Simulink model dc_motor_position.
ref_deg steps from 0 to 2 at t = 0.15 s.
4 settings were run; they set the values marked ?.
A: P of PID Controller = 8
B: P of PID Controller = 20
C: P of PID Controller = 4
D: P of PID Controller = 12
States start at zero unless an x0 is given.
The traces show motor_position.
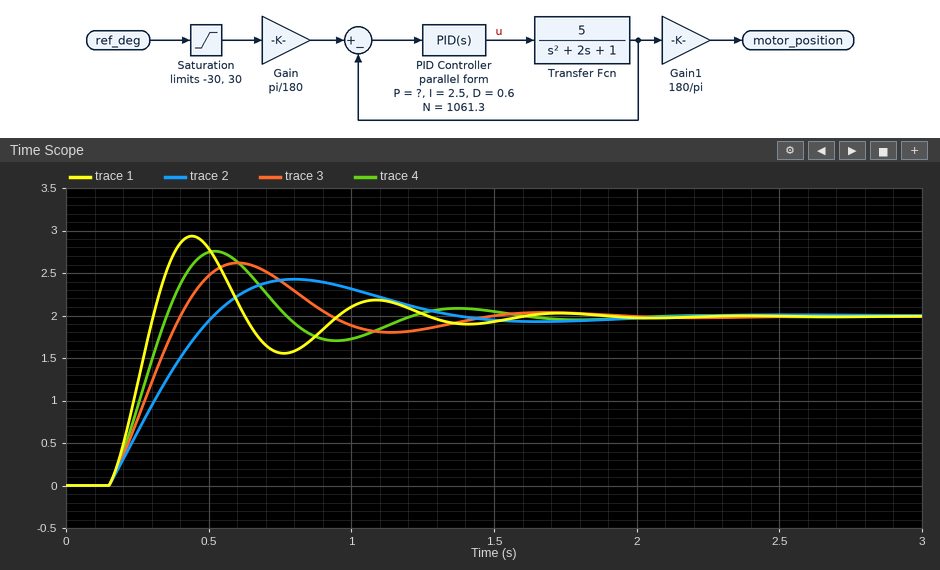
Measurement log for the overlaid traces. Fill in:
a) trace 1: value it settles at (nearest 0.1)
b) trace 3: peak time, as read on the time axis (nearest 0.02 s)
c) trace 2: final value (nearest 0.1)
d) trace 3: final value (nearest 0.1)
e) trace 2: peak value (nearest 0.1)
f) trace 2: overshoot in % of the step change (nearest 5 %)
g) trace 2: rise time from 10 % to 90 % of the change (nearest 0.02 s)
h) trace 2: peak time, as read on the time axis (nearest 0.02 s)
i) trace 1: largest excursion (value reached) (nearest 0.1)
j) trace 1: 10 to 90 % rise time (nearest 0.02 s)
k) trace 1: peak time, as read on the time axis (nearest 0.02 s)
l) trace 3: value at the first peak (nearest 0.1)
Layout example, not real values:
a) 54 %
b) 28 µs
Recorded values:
a) 2.0
b) 0.60 s
c) 2.0
d) 2.0
e) 2.4
f) 20 %
g) 0.28 s
h) 0.80 s
i) 2.9
j) 0.12 s
k) 0.44 s
l) 2.6
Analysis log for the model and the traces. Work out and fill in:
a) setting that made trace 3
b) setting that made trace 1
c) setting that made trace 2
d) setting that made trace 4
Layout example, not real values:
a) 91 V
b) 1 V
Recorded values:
a) A
b) B
c) C
d) D
